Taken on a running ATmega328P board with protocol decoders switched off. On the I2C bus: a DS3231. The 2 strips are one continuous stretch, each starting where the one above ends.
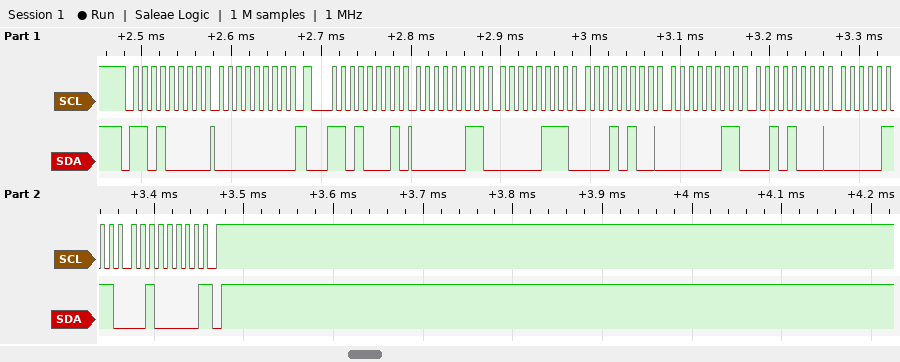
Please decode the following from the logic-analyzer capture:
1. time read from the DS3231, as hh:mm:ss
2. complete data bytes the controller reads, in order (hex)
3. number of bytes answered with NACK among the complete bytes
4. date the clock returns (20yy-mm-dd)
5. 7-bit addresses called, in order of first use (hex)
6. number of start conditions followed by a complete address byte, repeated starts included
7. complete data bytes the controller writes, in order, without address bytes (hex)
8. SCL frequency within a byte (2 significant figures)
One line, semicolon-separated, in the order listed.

14:07:03; 03 07 14 03 28 07 20; 1; 2020-07-28; 0x68; 2; 00; 100 kHz
